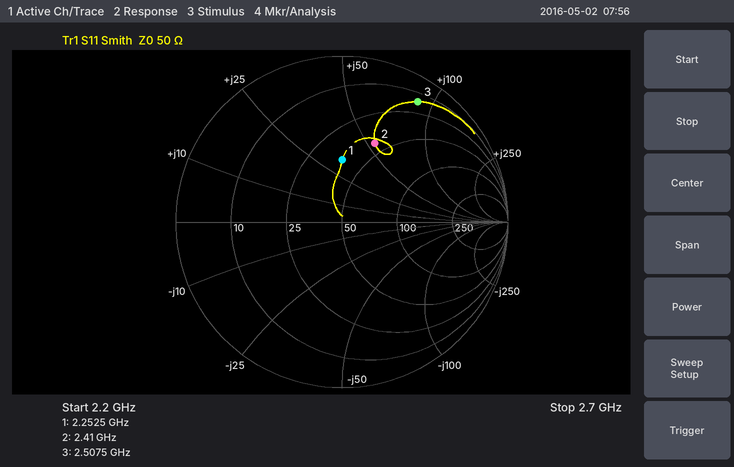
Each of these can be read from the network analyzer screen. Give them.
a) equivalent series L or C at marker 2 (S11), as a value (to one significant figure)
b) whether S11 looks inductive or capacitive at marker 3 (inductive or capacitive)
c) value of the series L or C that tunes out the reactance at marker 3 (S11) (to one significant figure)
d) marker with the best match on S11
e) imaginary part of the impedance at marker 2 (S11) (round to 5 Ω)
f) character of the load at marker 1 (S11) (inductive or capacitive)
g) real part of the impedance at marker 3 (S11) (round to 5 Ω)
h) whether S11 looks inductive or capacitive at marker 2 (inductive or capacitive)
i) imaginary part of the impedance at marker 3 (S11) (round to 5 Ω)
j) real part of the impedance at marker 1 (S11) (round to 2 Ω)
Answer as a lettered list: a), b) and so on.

a) 4 nH
b) inductive
c) 700 fF
d) marker 1
e) +55 Ω
f) inductive
g) 15 Ω
h) inductive
i) +90 Ω
j) 38 Ω
